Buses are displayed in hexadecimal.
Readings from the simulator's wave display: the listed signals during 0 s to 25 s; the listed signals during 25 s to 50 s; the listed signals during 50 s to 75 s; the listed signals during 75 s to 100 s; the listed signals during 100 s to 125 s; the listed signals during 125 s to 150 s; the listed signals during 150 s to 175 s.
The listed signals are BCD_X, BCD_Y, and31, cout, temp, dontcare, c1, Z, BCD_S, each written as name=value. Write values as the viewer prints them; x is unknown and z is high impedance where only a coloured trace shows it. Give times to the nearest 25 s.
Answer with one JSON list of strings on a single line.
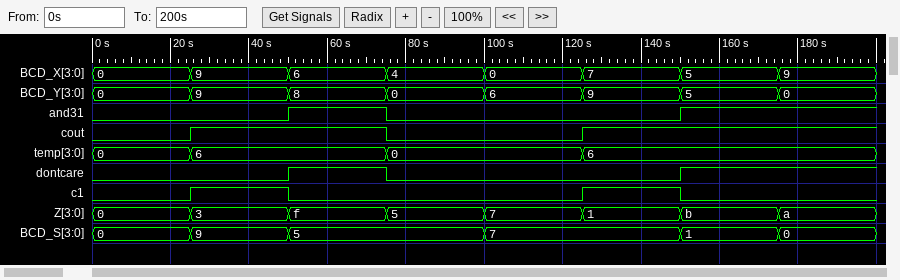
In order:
["BCD_X=0, BCD_Y=0, and31=0, cout=0, temp=0, dontcare=0, c1=0, Z=0, BCD_S=0", "BCD_X=9, BCD_Y=9, and31=0, cout=1, temp=6, dontcare=0, c1=1, Z=3, BCD_S=9", "BCD_X=6, BCD_Y=8, and31=1, cout=1, temp=6, dontcare=1, c1=0, Z=f, BCD_S=5", "BCD_X=4, BCD_Y=0, and31=0, cout=0, temp=0, dontcare=0, c1=0, Z=5, BCD_S=5", "BCD_X=0, BCD_Y=6, and31=0, cout=0, temp=0, dontcare=0, c1=0, Z=7, BCD_S=7", "BCD_X=7, BCD_Y=9, and31=0, cout=1, temp=6, dontcare=0, c1=1, Z=1, BCD_S=7", "BCD_X=5, BCD_Y=5, and31=1, cout=1, temp=6, dontcare=1, c1=0, Z=b, BCD_S=1"]
